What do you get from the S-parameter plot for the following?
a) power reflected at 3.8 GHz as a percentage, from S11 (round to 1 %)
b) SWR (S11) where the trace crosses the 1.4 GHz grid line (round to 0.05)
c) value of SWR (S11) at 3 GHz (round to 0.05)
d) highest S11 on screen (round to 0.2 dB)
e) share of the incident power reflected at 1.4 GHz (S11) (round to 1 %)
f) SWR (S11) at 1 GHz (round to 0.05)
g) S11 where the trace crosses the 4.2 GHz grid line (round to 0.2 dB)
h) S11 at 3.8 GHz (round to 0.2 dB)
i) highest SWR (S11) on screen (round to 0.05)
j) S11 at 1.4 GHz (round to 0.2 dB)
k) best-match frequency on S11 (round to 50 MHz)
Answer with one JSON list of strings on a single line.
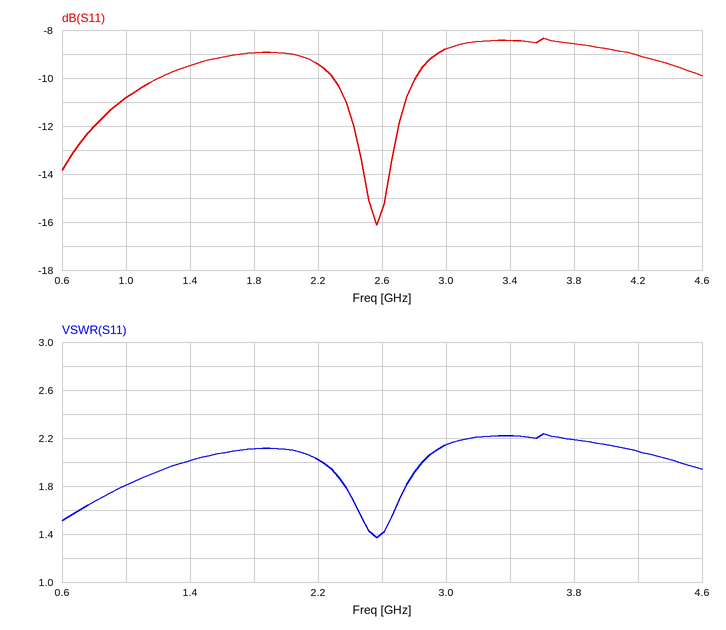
["14 %", "2.00", "2.15", "-8.4 dB", "11 %", "1.80", "-9.0 dB", "-8.6 dB", "2.25", "-9.4 dB", "2.55 GHz"]
